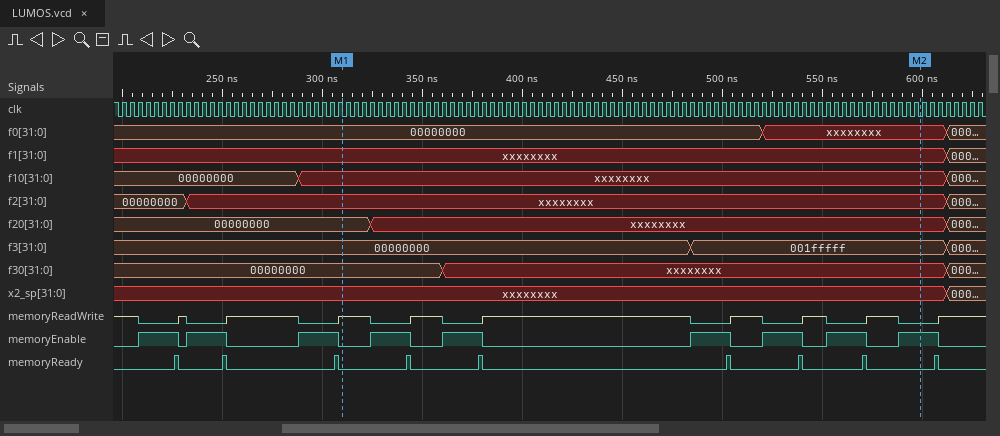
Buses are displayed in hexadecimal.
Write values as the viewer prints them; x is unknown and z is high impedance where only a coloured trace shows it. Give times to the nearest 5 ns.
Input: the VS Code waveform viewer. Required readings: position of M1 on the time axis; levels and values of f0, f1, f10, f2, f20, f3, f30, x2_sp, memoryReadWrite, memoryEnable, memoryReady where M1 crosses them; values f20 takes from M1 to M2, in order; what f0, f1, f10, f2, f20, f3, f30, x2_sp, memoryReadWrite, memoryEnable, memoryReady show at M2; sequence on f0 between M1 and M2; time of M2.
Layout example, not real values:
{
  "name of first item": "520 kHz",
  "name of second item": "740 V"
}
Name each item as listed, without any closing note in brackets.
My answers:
{
  "position of M1 on the time axis": "310 ns",
  "levels and values of f0, f1, f10, f2, f20, f3, f30, x2_sp, memoryReadWrite, memoryEnable, memoryReady where M1 crosses them": "f0=00000000, f1=xxxxxxxx, f10=xxxxxxxx, f2=xxxxxxxx, f20=00000000, f3=00000000, f30=00000000, x2_sp=xxxxxxxx, memoryReadWrite=z, memoryEnable=0, memoryReady=0",
  "values f20 takes from M1 to M2, in order": "00000000, xxxxxxxx",
  "what f0, f1, f10, f2, f20, f3, f30, x2_sp, memoryReadWrite, memoryEnable, memoryReady show at M2": "f0=xxxxxxxx, f1=xxxxxxxx, f10=xxxxxxxx, f2=xxxxxxxx, f20=xxxxxxxx, f3=001fffff, f30=xxxxxxxx, x2_sp=xxxxxxxx, memoryReadWrite=0, memoryEnable=1, memoryReady=0",
  "sequence on f0 between M1 and M2": "00000000, xxxxxxxx",
  "time of M2": "600 ns"
}
